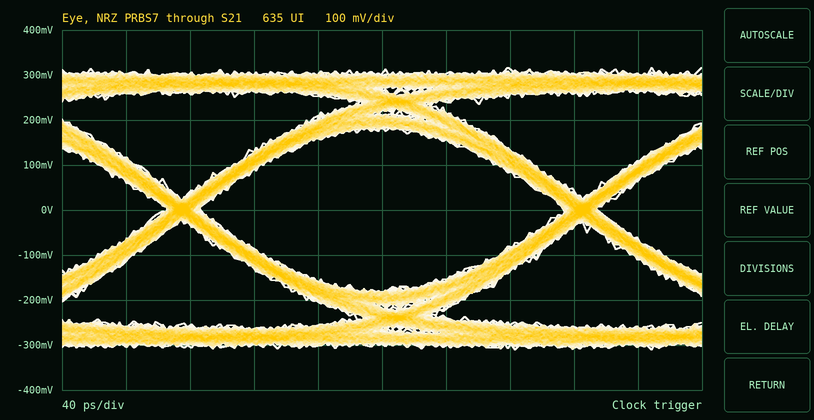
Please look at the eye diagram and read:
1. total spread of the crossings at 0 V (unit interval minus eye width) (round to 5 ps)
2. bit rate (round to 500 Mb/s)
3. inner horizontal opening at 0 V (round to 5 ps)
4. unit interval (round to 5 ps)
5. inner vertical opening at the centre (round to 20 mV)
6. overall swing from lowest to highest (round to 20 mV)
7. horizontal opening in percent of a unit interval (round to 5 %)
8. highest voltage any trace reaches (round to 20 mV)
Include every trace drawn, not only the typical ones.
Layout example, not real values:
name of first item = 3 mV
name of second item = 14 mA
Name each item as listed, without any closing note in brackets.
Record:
total spread of the crossings at 0 V (unit interval minus eye width) = 25 ps
bit rate = 4.0 Gb/s
inner horizontal opening at 0 V = 225 ps
unit interval = 250 ps
inner vertical opening at the centre = 360 mV
overall swing from lowest to highest = 620 mV
horizontal opening in percent of a unit interval = 90 %
highest voltage any trace reaches = 320 mV
